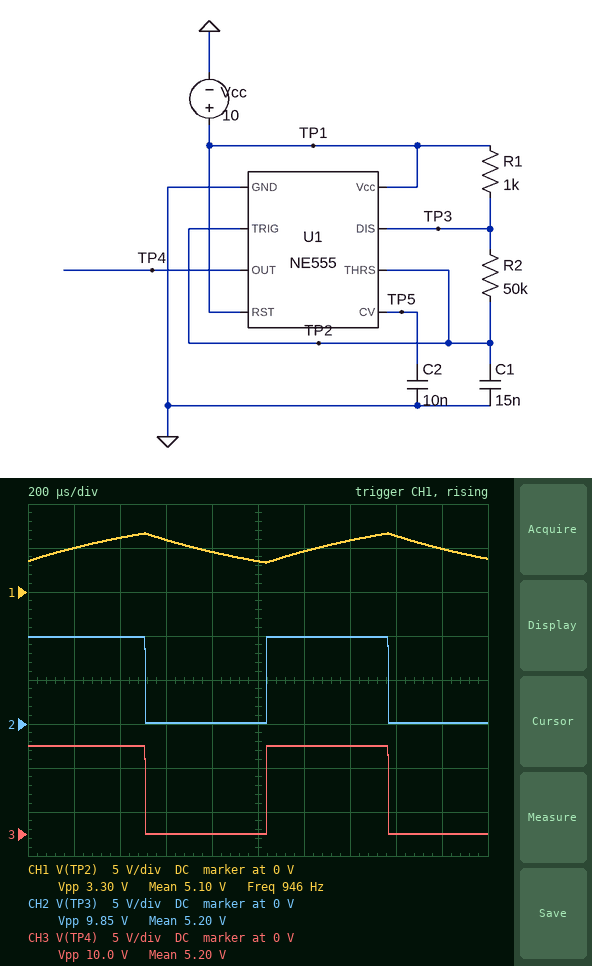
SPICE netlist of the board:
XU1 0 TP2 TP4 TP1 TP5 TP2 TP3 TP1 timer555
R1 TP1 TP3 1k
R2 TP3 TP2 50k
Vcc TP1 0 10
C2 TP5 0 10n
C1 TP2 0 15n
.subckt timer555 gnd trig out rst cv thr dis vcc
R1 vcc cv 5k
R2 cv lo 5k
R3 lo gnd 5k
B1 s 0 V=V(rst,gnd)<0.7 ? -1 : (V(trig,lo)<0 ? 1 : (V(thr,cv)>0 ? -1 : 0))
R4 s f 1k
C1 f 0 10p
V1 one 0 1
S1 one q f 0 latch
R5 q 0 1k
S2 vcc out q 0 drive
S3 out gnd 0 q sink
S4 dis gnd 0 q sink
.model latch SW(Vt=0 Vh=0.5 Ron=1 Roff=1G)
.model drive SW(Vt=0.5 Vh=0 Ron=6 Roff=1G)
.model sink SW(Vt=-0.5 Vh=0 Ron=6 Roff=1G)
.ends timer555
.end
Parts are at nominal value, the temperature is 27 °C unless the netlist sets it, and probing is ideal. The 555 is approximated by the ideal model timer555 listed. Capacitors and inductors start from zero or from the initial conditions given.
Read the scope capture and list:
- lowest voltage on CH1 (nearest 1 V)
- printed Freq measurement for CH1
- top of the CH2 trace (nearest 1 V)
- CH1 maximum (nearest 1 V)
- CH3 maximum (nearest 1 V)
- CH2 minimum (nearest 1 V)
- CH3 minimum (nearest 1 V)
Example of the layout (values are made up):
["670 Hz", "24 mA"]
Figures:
["3 V", "946 Hz", "10 V", "7 V", "10 V", "0 V", "0 V"]
